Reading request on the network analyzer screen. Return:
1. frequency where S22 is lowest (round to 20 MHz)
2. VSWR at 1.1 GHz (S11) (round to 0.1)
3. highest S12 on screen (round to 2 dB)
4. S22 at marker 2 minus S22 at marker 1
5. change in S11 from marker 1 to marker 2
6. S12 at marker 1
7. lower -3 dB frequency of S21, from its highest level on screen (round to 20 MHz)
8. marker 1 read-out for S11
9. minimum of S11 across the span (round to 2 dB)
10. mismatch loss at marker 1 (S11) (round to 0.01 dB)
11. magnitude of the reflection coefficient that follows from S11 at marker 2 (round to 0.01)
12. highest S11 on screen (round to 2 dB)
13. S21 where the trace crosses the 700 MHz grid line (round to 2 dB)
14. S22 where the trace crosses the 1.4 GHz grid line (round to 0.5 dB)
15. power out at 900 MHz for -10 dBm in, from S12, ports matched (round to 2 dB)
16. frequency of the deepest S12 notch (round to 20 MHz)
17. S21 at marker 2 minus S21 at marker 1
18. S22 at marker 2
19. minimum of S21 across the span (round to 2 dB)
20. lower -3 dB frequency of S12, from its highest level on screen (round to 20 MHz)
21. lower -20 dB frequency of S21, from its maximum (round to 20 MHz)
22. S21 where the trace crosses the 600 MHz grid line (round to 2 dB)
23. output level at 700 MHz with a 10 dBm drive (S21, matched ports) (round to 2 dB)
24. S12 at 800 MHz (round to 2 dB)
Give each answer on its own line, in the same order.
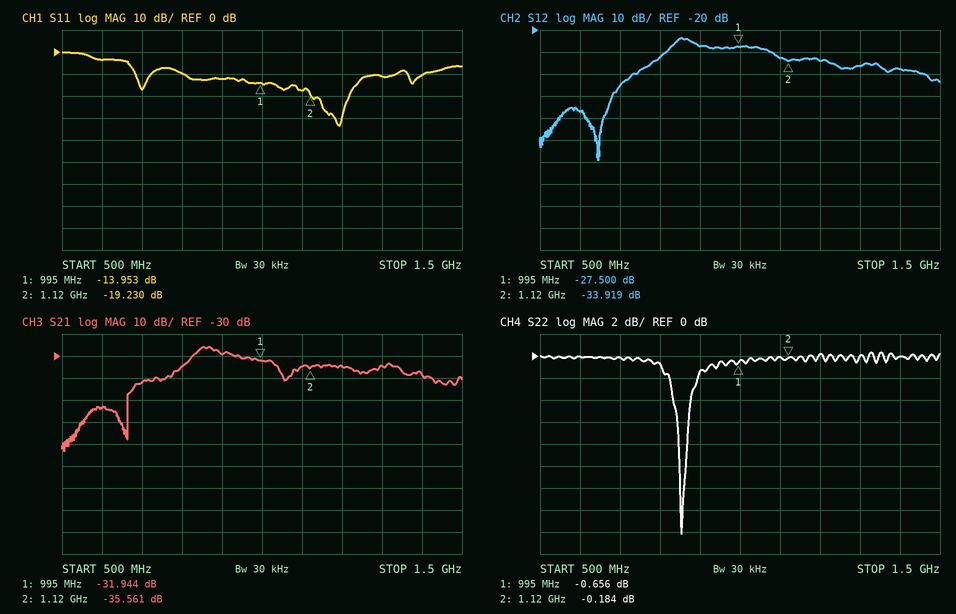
860 MHz
1.3
-24 dB
0.472 dB
-5.277 dB
-27.500 dB
840 MHz
-13.953 dB
-34 dB
0.18 dB
0.11
0 dB
-42 dB
0.0 dB
-38 dBm
640 MHz
-3.617 dB
-0.184 dB
-74 dB
840 MHz
680 MHz
-54 dB
-32 dBm
-32 dB
